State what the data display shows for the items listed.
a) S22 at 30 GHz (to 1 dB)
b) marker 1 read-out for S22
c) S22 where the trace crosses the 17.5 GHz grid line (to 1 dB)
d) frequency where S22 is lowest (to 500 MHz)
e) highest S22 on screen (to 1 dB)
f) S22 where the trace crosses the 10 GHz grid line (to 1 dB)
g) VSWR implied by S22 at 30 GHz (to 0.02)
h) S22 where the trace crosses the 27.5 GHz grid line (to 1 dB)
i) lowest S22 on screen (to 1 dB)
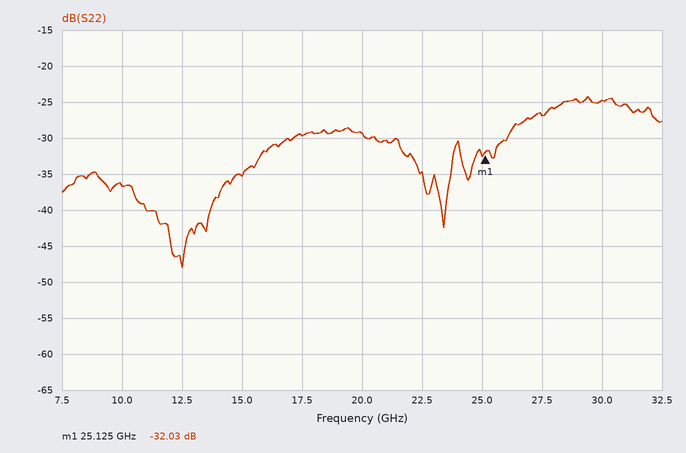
-25 dB
-32.03 dB
-30 dB
12.5 GHz
-24 dB
-37 dB
1.12
-27 dB
-48 dB
